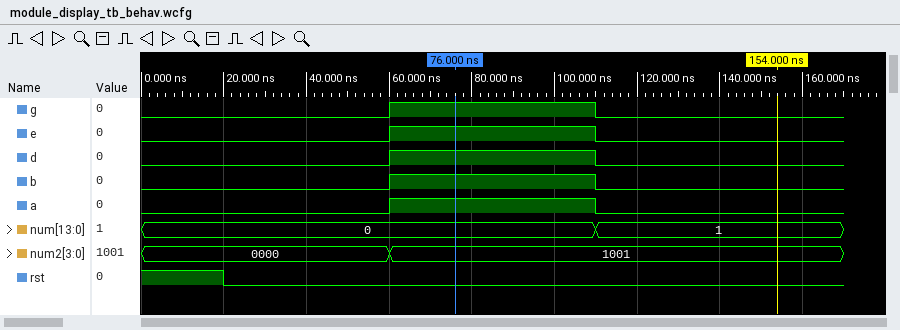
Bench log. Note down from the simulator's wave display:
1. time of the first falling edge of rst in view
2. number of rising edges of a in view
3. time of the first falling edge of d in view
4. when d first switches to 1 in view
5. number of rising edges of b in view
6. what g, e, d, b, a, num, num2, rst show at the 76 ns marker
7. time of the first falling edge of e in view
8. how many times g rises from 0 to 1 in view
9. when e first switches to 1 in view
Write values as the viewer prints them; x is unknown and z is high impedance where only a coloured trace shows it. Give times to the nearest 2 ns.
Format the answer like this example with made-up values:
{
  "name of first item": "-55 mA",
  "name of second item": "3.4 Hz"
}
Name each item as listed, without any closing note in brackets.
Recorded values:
{
  "time of the first falling edge of rst in view": "20 ns",
  "number of rising edges of a in view": "1",
  "time of the first falling edge of d in view": "110 ns",
  "when d first switches to 1 in view": "60 ns",
  "number of rising edges of b in view": "1",
  "what g, e, d, b, a, num, num2, rst show at the 76 ns marker": "g=1, e=1, d=1, b=1, a=1, num=0, num2=1001, rst=0",
  "time of the first falling edge of e in view": "110 ns",
  "how many times g rises from 0 to 1 in view": "1",
  "when e first switches to 1 in view": "60 ns"
}
